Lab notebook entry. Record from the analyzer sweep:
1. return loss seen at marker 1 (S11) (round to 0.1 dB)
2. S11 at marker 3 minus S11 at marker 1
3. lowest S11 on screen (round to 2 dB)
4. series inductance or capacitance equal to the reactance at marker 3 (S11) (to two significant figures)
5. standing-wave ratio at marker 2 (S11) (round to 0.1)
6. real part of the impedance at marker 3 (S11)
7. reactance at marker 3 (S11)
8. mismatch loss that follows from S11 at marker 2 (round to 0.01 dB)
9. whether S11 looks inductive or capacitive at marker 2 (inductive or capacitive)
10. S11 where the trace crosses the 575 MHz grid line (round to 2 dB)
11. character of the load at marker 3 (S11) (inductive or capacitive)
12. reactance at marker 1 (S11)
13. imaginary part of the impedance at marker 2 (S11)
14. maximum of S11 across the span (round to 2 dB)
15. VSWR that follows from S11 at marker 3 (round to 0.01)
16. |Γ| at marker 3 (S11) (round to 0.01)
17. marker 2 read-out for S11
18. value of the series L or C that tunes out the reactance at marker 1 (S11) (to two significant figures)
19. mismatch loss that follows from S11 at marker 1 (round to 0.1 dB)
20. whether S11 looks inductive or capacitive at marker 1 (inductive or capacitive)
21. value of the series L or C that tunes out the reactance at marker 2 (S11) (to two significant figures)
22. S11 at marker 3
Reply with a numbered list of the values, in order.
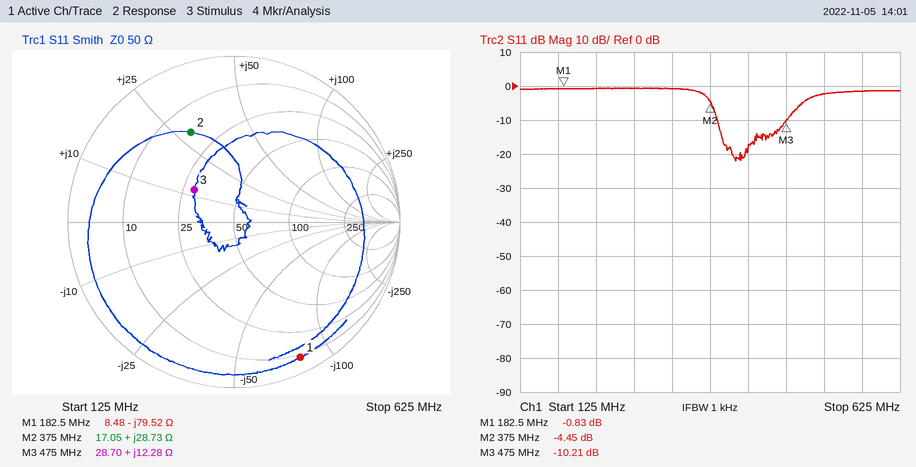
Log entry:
1. 0.8 dB
2. -9.38 dB
3. -22 dB
4. 4.1 nH
5. 4.0
6. 28.70 Ω
7. +12.28 Ω
8. 1.93 dB
9. inductive
10. -2 dB
11. inductive
12. -79.52 Ω
13. +28.73 Ω
14. 0 dB
15. 1.89
16. 0.31
17. -4.45 dB
18. 69 nH
19. 7.6 dB
20. capacitive
21. 15 pF
22. -10.21 dB
